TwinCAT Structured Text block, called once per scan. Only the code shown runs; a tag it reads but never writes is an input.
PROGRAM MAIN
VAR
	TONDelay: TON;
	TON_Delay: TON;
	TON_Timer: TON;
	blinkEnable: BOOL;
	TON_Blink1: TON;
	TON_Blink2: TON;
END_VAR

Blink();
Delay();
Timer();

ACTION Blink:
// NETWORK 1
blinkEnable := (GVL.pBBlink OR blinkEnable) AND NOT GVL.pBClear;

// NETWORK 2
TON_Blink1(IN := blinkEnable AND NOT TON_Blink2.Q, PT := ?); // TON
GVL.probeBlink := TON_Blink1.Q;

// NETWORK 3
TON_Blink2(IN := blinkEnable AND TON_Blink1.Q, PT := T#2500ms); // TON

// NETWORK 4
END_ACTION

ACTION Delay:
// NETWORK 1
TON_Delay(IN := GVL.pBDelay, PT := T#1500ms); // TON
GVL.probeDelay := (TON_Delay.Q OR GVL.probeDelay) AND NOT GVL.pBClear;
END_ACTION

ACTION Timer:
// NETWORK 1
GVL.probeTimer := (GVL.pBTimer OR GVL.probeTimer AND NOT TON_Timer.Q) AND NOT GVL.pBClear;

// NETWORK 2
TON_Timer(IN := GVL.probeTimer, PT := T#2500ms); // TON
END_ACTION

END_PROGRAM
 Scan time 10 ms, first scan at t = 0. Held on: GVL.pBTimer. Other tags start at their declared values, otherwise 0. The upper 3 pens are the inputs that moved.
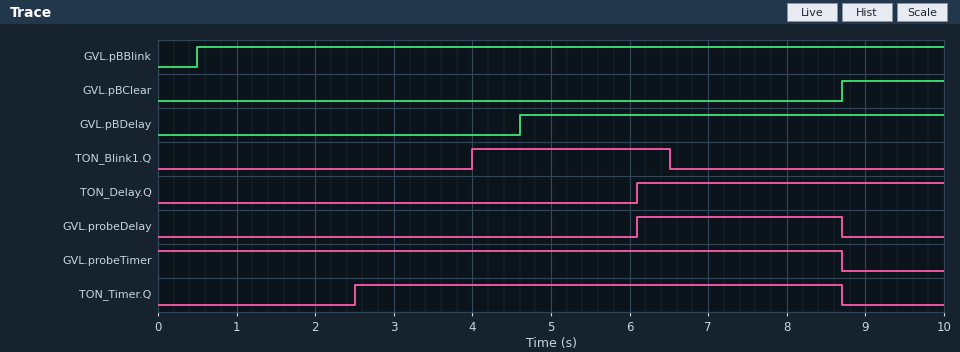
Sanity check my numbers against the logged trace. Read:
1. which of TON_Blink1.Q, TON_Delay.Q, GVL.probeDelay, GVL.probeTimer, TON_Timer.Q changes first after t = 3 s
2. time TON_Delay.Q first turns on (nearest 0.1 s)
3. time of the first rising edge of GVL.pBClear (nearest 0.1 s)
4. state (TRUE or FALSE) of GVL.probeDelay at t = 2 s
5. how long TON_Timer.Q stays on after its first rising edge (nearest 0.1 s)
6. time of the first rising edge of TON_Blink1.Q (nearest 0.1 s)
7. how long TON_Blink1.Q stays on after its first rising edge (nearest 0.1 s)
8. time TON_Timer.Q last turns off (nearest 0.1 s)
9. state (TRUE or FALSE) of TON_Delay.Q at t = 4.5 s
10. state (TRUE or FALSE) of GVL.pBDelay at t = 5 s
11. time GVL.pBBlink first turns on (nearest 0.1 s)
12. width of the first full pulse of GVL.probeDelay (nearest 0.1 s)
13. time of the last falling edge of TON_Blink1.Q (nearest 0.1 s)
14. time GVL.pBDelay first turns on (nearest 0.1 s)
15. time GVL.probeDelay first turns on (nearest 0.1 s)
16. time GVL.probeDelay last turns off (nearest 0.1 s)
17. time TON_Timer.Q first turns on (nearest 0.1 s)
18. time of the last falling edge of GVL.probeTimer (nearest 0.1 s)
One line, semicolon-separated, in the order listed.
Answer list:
TON_Blink1.Q; 6.1 s; 8.7 s; FALSE; 6.2 s; 4.0 s; 2.5 s; 8.7 s; FALSE; TRUE; 0.5 s; 2.6 s; 6.5 s; 4.6 s; 6.1 s; 8.7 s; 2.5 s; 8.7 s
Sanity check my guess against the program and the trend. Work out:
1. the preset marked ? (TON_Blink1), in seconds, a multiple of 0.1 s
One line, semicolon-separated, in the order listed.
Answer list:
3.5 s
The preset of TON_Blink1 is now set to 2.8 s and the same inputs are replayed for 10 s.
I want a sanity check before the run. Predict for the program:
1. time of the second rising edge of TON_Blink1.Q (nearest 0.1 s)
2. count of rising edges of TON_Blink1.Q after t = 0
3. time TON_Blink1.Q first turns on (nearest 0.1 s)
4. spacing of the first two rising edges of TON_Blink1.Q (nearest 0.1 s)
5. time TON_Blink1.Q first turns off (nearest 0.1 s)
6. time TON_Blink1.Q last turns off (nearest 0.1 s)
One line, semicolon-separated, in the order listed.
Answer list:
8.6 s; 2; 3.3 s; 5.3 s; 5.8 s; 8.7 s
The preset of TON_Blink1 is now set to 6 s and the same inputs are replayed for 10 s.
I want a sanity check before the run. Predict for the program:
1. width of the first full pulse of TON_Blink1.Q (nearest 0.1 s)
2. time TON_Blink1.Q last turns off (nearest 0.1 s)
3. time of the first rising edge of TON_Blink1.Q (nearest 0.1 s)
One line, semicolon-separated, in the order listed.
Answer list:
2.2 s; 8.7 s; 6.5 s
